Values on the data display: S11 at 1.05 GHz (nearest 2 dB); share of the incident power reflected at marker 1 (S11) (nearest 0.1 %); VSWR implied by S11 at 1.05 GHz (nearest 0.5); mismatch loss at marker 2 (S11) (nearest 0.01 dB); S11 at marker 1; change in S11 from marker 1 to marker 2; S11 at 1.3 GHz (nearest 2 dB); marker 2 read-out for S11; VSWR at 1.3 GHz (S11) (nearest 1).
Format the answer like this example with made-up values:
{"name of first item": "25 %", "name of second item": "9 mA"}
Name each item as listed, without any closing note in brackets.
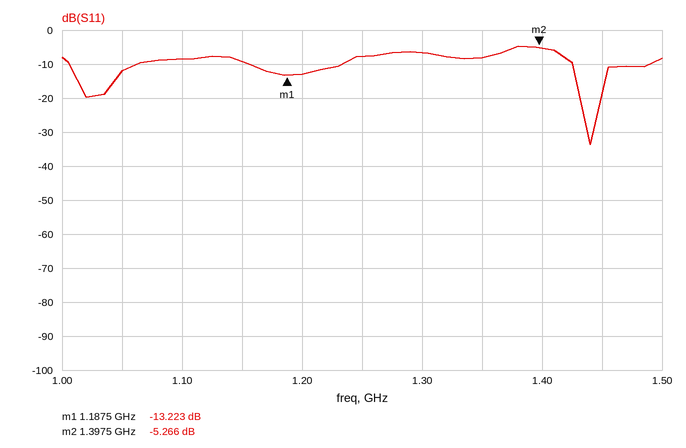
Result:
{"S11 at 1.05 GHz": "-12 dB", "share of the incident power reflected at marker 1 (S11)": "4.8 %", "VSWR implied by S11 at 1.05 GHz": "1.5", "mismatch loss at marker 2 (S11)": "1.53 dB", "S11 at marker 1": "-13.223 dB", "change in S11 from marker 1 to marker 2": "7.957 dB", "S11 at 1.3 GHz": "-6 dB", "marker 2 read-out for S11": "-5.266 dB", "VSWR at 1.3 GHz (S11)": "3"}
